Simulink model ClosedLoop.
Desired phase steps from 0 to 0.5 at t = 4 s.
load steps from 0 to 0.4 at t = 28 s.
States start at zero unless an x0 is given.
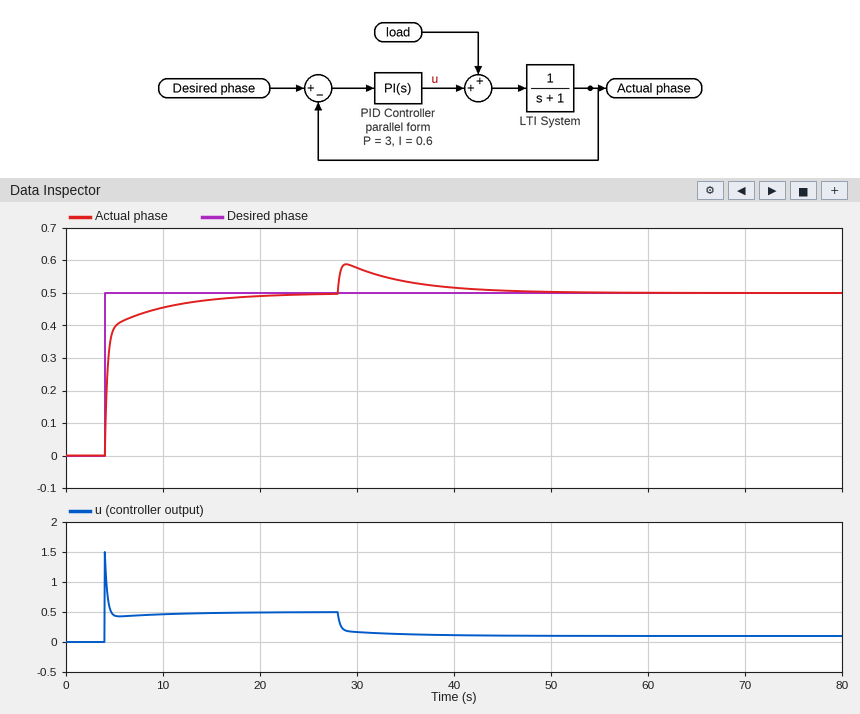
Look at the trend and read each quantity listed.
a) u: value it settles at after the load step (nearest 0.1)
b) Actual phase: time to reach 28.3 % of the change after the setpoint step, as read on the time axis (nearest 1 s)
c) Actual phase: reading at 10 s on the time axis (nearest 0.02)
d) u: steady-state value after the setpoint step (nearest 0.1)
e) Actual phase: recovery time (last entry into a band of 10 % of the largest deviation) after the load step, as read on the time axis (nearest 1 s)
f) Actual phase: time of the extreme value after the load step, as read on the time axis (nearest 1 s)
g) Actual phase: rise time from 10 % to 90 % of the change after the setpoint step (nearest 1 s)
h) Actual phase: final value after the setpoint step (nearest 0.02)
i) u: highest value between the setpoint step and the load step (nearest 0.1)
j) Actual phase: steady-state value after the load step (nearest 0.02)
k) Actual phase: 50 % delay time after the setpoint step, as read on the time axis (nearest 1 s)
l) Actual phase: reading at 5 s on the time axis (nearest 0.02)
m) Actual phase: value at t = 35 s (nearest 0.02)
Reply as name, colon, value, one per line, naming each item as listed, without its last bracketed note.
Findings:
u: value it settles at after the load step: 0.1
Actual phase: time to reach 28.3 % of the change after the setpoint step, as read on the time axis: 4 s
Actual phase: reading at 10 s on the time axis: 0.46
u: steady-state value after the setpoint step: 0.5
Actual phase: recovery time (last entry into a band of 10 % of the largest deviation) after the load step, as read on the time axis: 44 s
Actual phase: time of the extreme value after the load step, as read on the time axis: 29 s
Actual phase: rise time from 10 % to 90 % of the change after the setpoint step: 5 s
Actual phase: final value after the setpoint step: 0.50
u: highest value between the setpoint step and the load step: 1.5
Actual phase: steady-state value after the load step: 0.50
Actual phase: 50 % delay time after the setpoint step, as read on the time axis: 4 s
Actual phase: reading at 5 s on the time axis: 0.40
Actual phase: value at t = 35 s: 0.54
